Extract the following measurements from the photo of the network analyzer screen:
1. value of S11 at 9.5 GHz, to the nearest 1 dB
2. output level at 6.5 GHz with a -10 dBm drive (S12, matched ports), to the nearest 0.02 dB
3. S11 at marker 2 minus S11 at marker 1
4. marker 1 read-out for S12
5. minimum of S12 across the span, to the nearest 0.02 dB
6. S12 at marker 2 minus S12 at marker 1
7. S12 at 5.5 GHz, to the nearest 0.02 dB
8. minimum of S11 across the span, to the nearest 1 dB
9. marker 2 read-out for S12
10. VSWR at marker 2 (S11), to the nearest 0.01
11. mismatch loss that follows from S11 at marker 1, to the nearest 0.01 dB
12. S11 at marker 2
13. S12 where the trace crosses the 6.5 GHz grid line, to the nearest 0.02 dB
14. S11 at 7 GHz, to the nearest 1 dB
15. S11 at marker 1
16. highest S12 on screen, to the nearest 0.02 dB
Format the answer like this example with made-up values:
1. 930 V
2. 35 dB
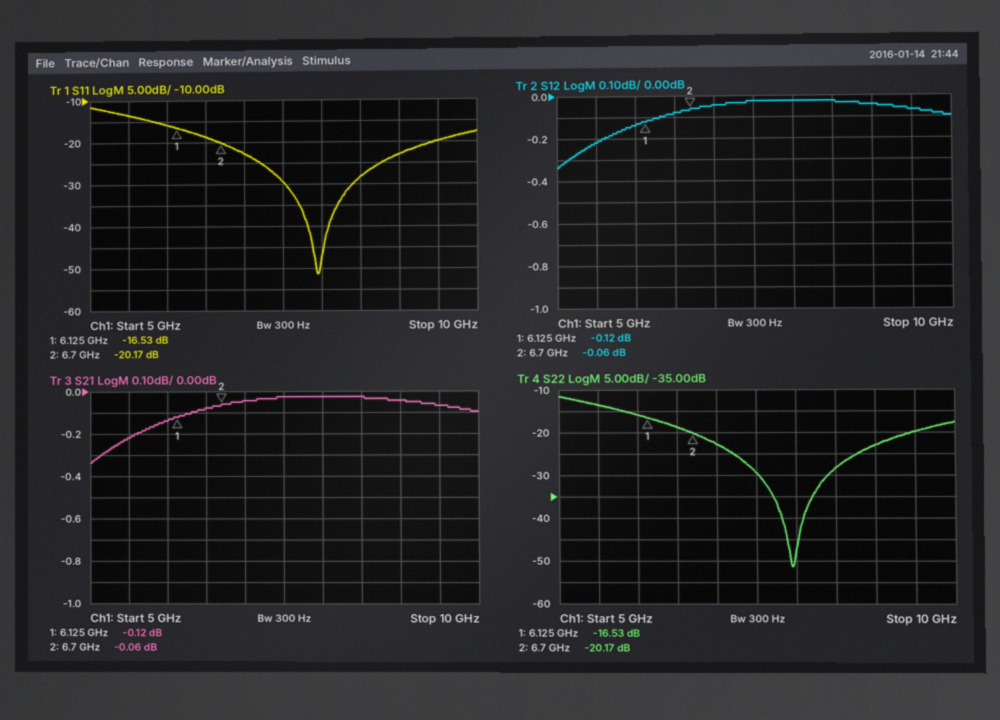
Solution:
1. -20 dB
2. -10.08 dBm
3. -3.64 dB
4. -0.12 dB
5. -0.34 dB
6. 0.06 dB
7. -0.22 dB
8. -51 dB
9. -0.06 dB
10. 1.22
11. 0.10 dB
12. -20.17 dB
13. -0.08 dB
14. -23 dB
15. -16.53 dB
16. -0.02 dB
